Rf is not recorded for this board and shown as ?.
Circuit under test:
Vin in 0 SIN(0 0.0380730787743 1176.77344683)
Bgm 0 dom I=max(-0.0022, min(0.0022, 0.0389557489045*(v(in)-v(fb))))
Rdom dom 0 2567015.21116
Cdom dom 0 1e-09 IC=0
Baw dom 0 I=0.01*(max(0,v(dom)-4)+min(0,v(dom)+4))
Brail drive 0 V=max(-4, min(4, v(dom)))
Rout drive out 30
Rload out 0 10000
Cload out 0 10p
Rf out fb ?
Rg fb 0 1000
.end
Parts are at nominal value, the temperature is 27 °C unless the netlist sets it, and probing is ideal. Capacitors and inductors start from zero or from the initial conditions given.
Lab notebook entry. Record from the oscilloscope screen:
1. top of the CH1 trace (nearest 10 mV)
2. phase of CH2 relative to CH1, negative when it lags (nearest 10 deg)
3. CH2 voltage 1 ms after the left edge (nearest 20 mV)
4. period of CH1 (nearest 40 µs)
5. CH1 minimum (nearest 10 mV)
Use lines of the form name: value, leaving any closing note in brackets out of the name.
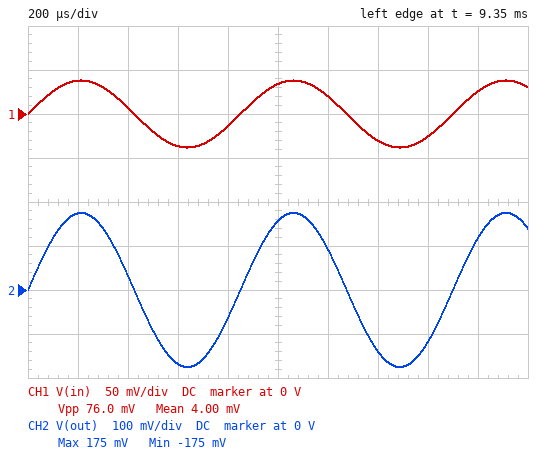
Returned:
top of the CH1 trace: 40 mV
phase of CH2 relative to CH1, negative when it lags: 0 deg
CH2 voltage 1 ms after the left edge: 160 mV
period of CH1: 840 µs
CH1 minimum: -40 mV
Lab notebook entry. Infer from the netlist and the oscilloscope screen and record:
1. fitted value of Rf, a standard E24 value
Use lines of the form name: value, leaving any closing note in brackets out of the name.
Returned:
fitted value of Rf, a standard E24 value: 3.6 kΩ
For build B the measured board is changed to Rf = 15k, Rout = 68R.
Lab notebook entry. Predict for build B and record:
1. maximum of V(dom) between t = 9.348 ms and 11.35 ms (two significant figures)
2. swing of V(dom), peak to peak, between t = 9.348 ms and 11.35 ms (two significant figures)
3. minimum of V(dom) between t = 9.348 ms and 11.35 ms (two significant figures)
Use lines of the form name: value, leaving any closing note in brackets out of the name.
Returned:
maximum of V(dom) between t = 9.348 ms and 11.35 ms: 620 mV
swing of V(dom), peak to peak, between t = 9.348 ms and 11.35 ms: 1.2 V
minimum of V(dom) between t = 9.348 ms and 11.35 ms: -620 mV
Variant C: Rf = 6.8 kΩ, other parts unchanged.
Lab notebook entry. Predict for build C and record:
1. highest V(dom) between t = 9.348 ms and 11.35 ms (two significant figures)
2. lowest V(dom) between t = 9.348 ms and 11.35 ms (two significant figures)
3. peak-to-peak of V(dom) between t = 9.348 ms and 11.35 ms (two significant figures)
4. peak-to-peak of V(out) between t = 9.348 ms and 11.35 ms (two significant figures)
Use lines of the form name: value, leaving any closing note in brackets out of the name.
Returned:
highest V(dom) between t = 9.348 ms and 11.35 ms: 300 mV
lowest V(dom) between t = 9.348 ms and 11.35 ms: -300 mV
peak-to-peak of V(dom) between t = 9.348 ms and 11.35 ms: 600 mV
peak-to-peak of V(out) between t = 9.348 ms and 11.35 ms: 590 mV
